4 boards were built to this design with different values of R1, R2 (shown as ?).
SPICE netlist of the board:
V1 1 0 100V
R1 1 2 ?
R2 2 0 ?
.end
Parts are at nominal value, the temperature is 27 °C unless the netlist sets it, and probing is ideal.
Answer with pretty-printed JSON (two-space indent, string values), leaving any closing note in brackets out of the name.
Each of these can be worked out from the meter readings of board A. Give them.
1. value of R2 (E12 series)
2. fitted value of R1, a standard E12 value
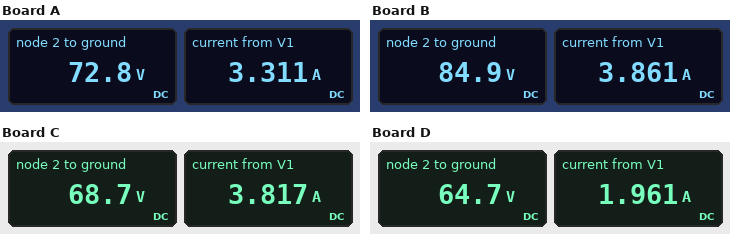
{
  "value of R2": "22 Ω",
  "fitted value of R1, a standard E12 value": "8.2 Ω"
}
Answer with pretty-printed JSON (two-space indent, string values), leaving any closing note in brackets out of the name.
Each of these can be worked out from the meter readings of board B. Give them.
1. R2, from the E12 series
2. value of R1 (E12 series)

{
  "R2, from the E12 series": "22 Ω",
  "value of R1": "3.9 Ω"
}
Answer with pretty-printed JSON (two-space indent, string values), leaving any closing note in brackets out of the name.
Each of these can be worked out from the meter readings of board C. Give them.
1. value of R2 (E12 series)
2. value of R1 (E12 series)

{
  "value of R2": "18 Ω",
  "value of R1": "8.2 Ω"
}
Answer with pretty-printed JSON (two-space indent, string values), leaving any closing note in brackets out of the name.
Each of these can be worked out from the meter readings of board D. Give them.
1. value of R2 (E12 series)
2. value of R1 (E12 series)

{
  "value of R2": "33 Ω",
  "value of R1": "18 Ω"
}
